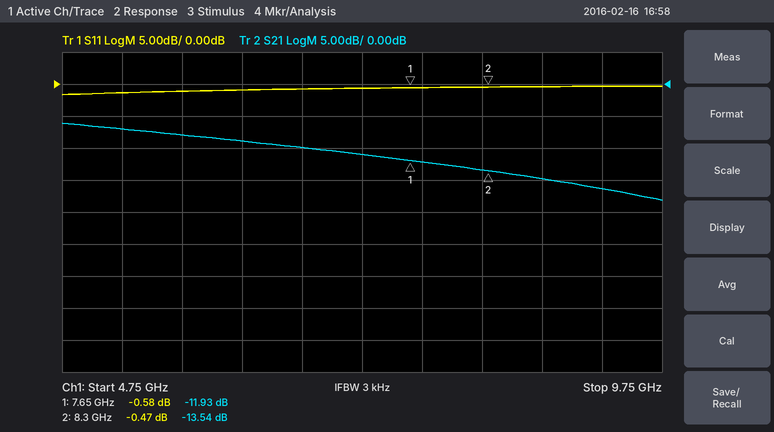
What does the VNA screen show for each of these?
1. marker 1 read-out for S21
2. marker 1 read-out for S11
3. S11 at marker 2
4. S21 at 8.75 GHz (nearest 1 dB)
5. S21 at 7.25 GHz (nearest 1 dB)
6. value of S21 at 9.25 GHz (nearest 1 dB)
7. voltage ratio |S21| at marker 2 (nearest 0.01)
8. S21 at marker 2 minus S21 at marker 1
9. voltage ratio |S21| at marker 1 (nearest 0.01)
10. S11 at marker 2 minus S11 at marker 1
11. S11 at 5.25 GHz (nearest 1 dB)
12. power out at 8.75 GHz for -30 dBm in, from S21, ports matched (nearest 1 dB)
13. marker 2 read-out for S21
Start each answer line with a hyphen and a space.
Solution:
- -11.93 dB
- -0.58 dB
- -0.47 dB
- -15 dB
- -11 dB
- -16 dB
- 0.21
- -1.61 dB
- 0.25
- 0.11 dB
- -1 dB
- -45 dBm
- -13.54 dB
